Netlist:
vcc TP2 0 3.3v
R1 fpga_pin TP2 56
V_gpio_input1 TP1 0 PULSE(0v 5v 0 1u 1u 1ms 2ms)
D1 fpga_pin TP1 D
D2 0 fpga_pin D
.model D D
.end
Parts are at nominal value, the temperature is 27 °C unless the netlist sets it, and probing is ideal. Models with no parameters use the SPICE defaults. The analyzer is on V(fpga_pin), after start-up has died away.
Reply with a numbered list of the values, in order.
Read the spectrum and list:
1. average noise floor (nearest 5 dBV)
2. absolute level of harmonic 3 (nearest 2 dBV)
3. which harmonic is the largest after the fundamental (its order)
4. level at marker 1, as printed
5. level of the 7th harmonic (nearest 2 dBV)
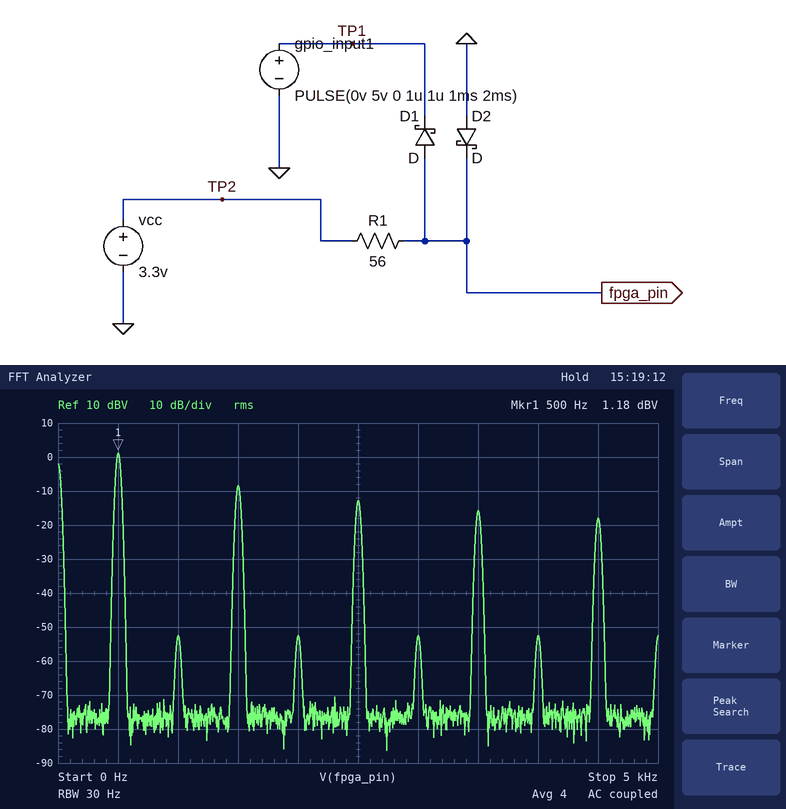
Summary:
1. -75 dBV
2. -8 dBV
3. 3
4. 1.18 dBV
5. -16 dBV
